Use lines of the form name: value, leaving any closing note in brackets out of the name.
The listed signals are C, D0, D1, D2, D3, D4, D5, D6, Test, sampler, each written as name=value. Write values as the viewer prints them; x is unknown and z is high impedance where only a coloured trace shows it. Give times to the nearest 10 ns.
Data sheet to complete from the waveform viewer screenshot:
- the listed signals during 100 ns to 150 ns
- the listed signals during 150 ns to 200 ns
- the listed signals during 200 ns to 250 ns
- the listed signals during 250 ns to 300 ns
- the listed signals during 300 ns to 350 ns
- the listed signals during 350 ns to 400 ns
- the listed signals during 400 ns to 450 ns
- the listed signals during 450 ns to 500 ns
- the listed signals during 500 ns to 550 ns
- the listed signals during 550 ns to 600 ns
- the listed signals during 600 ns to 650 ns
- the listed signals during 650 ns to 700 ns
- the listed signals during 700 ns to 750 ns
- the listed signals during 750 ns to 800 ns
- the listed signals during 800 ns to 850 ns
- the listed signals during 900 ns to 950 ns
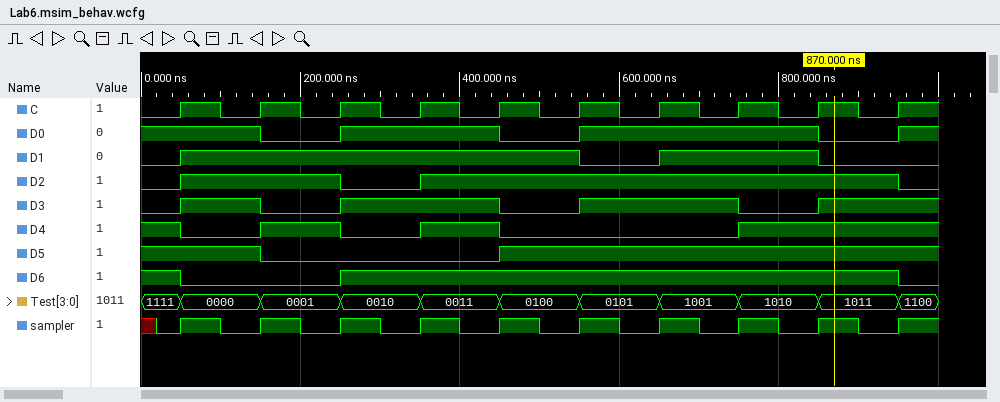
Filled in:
the listed signals during 100 ns to 150 ns: C=0, D0=1, D1=1, D2=1, D3=1, D4=0, D5=1, D6=0, Test=0000, sampler=0
the listed signals during 150 ns to 200 ns: C=1, D0=0, D1=1, D2=1, D3=0, D4=1, D5=0, D6=0, Test=0001, sampler=1
the listed signals during 200 ns to 250 ns: C=0, D0=0, D1=1, D2=1, D3=0, D4=1, D5=0, D6=0, Test=0001, sampler=0
the listed signals during 250 ns to 300 ns: C=1, D0=1, D1=1, D2=0, D3=1, D4=0, D5=0, D6=1, Test=0010, sampler=1
the listed signals during 300 ns to 350 ns: C=0, D0=1, D1=1, D2=0, D3=1, D4=0, D5=0, D6=1, Test=0010, sampler=0
the listed signals during 350 ns to 400 ns: C=1, D0=1, D1=1, D2=1, D3=1, D4=1, D5=0, D6=1, Test=0011, sampler=1
the listed signals during 400 ns to 450 ns: C=0, D0=1, D1=1, D2=1, D3=1, D4=1, D5=0, D6=1, Test=0011, sampler=0
the listed signals during 450 ns to 500 ns: C=1, D0=0, D1=1, D2=1, D3=0, D4=0, D5=1, D6=1, Test=0100, sampler=1
the listed signals during 500 ns to 550 ns: C=0, D0=0, D1=1, D2=1, D3=0, D4=0, D5=1, D6=1, Test=0100, sampler=0
the listed signals during 550 ns to 600 ns: C=1, D0=1, D1=0, D2=1, D3=1, D4=0, D5=1, D6=1, Test=0101, sampler=1
the listed signals during 600 ns to 650 ns: C=0, D0=1, D1=0, D2=1, D3=1, D4=0, D5=1, D6=1, Test=0101, sampler=0
the listed signals during 650 ns to 700 ns: C=1, D0=1, D1=1, D2=1, D3=1, D4=0, D5=1, D6=1, Test=1001, sampler=1
the listed signals during 700 ns to 750 ns: C=0, D0=1, D1=1, D2=1, D3=1, D4=0, D5=1, D6=1, Test=1001, sampler=0
the listed signals during 750 ns to 800 ns: C=1, D0=1, D1=1, D2=1, D3=0, D4=1, D5=1, D6=1, Test=1010, sampler=1
the listed signals during 800 ns to 850 ns: C=0, D0=1, D1=1, D2=1, D3=0, D4=1, D5=1, D6=1, Test=1010, sampler=0
the listed signals during 900 ns to 950 ns: C=0, D0=0, D1=0, D2=1, D3=1, D4=1, D5=1, D6=1, Test=1011, sampler=0
